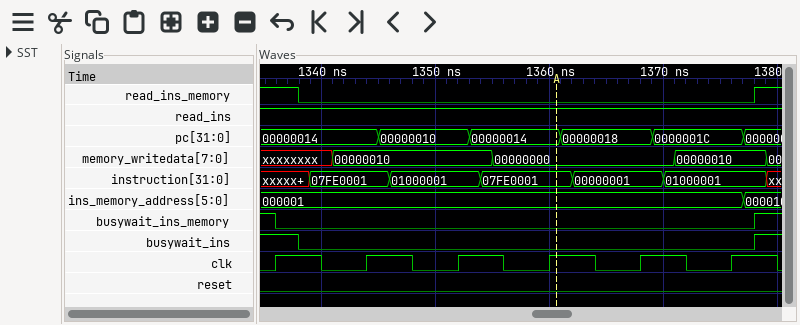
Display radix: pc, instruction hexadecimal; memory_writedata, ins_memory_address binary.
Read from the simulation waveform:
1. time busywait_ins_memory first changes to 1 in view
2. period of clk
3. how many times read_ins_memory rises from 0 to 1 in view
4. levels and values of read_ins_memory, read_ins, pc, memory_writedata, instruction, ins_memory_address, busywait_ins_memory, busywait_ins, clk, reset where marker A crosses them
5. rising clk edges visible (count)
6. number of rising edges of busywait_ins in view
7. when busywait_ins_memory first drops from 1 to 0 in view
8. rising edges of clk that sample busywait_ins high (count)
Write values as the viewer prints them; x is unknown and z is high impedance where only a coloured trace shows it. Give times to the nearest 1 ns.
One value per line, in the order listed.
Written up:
1378 ns
8 ns
1
read_ins_memory=0, read_ins=1, pc=00000014, memory_writedata=00000000, instruction=07FE0001, ins_memory_address=000001, busywait_ins_memory=0, busywait_ins=0, clk=1, reset=0
6
1
1336 ns
1
